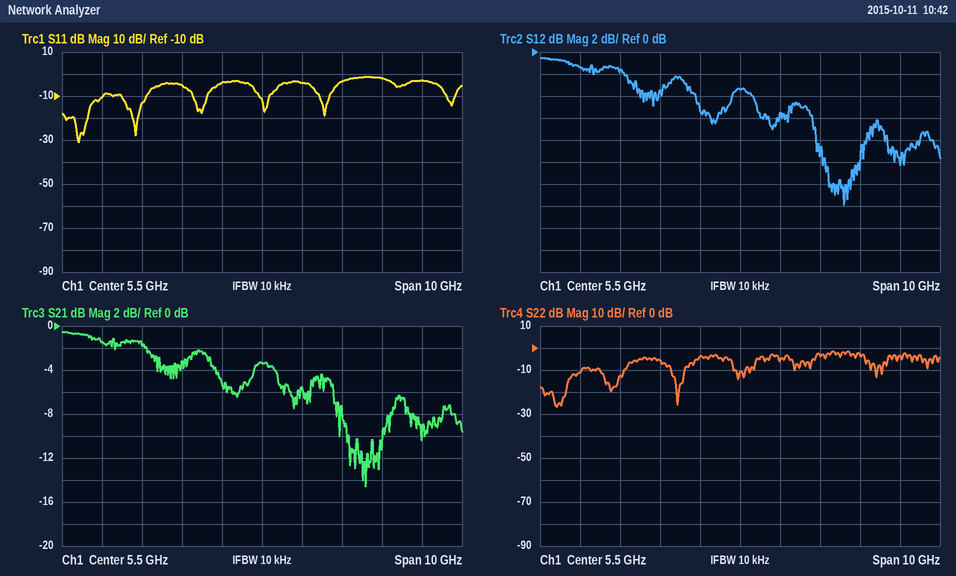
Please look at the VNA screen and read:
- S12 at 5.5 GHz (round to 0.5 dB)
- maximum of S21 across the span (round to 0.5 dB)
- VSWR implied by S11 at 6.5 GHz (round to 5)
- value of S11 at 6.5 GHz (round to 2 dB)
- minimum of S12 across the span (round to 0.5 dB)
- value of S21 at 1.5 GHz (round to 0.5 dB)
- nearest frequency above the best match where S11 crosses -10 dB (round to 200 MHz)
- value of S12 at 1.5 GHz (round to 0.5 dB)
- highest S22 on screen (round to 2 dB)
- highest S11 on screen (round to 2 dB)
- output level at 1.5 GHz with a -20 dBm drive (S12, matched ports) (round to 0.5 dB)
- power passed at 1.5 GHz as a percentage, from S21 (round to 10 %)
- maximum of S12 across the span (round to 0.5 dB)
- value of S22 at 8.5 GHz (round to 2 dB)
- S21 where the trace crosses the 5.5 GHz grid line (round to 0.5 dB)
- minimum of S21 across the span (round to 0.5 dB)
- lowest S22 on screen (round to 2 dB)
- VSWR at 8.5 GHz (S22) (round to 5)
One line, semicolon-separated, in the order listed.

-3.5 dB; -0.5 dB; 5; -4 dB; -14.0 dB; -1.5 dB; 1.6 GHz; -1.5 dB; -2 dB; -2 dB; -21.5 dBm; 70 %; -0.5 dB; -4 dB; -3.5 dB; -14.5 dB; -26 dB; 5
